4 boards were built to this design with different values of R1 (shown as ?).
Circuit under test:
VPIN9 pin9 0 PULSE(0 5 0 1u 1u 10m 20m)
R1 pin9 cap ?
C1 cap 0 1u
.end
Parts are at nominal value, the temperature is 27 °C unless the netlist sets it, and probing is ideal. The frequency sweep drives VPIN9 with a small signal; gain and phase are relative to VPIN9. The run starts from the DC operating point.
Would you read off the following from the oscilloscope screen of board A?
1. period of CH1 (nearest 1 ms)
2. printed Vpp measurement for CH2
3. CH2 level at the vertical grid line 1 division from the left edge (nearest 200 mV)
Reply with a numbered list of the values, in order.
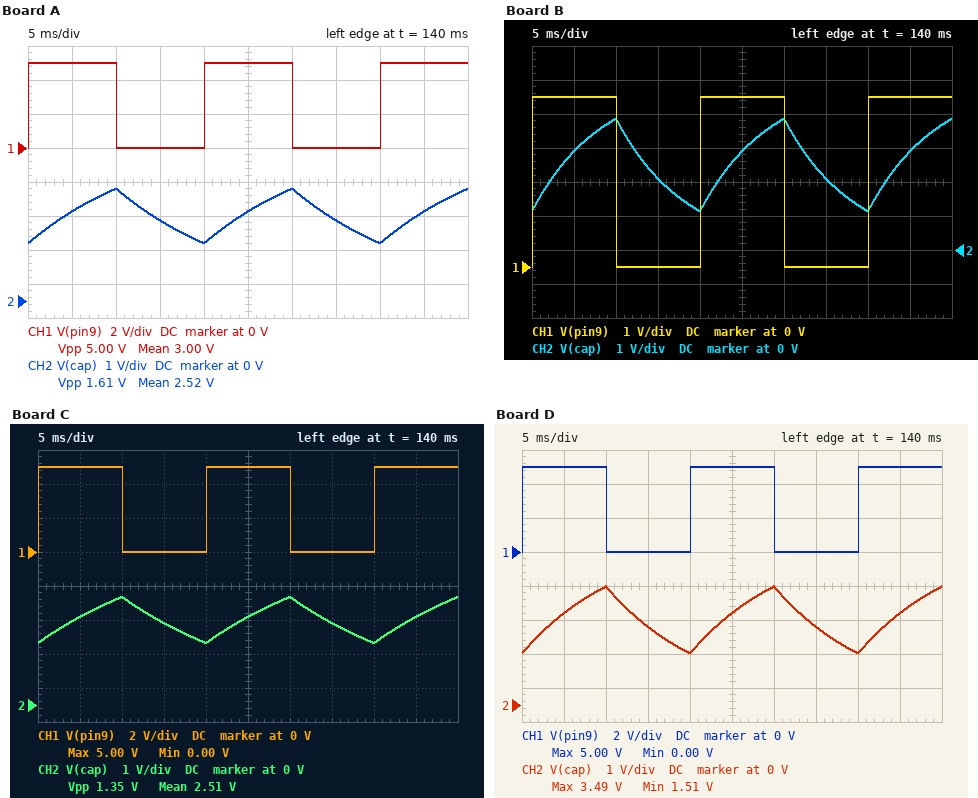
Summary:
1. 20 ms
2. 1.61 V
3. 2.6 V
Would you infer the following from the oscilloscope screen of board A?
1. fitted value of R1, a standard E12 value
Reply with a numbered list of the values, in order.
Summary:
1. 15 kΩ
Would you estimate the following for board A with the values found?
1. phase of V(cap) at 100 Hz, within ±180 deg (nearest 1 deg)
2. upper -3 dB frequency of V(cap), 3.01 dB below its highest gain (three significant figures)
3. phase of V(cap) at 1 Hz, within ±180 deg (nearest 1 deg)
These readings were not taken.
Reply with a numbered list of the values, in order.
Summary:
1. -84 deg
2. 10.6 Hz
3. -5 deg
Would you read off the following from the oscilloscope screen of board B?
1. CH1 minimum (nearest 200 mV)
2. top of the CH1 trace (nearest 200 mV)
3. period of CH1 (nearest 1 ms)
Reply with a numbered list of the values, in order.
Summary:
1. 0 V
2. 5.0 V
3. 20 ms
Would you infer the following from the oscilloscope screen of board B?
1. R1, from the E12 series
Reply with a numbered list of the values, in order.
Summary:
1. 8.2 kΩ
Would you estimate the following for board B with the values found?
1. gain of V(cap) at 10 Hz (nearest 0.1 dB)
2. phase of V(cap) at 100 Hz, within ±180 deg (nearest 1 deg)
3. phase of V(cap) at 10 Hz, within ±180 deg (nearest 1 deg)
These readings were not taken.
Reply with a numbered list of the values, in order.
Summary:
1. -1.0 dB
2. -79 deg
3. -27 deg
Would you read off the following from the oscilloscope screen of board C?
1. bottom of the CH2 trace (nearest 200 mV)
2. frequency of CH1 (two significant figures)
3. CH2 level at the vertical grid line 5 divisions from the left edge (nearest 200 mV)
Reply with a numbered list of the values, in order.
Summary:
1. 1.8 V
2. 50 Hz
3. 2.6 V
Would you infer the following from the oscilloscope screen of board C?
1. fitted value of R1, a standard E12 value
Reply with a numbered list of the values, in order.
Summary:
1. 18 kΩ
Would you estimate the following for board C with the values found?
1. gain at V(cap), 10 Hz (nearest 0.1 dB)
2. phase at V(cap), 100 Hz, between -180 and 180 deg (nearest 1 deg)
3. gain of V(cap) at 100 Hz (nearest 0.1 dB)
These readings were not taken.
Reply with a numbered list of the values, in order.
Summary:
1. -3.6 dB
2. -85 deg
3. -21.1 dB
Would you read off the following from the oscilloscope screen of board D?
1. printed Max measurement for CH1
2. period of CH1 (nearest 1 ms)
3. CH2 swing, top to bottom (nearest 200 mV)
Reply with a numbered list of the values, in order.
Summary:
1. 5.00 V
2. 20 ms
3. 2.0 V
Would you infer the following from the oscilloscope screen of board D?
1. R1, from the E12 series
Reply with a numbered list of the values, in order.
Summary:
1. 12 kΩ
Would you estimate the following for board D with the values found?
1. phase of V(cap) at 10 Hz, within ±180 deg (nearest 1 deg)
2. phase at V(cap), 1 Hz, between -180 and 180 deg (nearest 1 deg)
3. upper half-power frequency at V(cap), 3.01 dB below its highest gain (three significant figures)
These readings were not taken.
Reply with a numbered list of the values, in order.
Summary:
1. -37 deg
2. -4 deg
3. 13.3 Hz
